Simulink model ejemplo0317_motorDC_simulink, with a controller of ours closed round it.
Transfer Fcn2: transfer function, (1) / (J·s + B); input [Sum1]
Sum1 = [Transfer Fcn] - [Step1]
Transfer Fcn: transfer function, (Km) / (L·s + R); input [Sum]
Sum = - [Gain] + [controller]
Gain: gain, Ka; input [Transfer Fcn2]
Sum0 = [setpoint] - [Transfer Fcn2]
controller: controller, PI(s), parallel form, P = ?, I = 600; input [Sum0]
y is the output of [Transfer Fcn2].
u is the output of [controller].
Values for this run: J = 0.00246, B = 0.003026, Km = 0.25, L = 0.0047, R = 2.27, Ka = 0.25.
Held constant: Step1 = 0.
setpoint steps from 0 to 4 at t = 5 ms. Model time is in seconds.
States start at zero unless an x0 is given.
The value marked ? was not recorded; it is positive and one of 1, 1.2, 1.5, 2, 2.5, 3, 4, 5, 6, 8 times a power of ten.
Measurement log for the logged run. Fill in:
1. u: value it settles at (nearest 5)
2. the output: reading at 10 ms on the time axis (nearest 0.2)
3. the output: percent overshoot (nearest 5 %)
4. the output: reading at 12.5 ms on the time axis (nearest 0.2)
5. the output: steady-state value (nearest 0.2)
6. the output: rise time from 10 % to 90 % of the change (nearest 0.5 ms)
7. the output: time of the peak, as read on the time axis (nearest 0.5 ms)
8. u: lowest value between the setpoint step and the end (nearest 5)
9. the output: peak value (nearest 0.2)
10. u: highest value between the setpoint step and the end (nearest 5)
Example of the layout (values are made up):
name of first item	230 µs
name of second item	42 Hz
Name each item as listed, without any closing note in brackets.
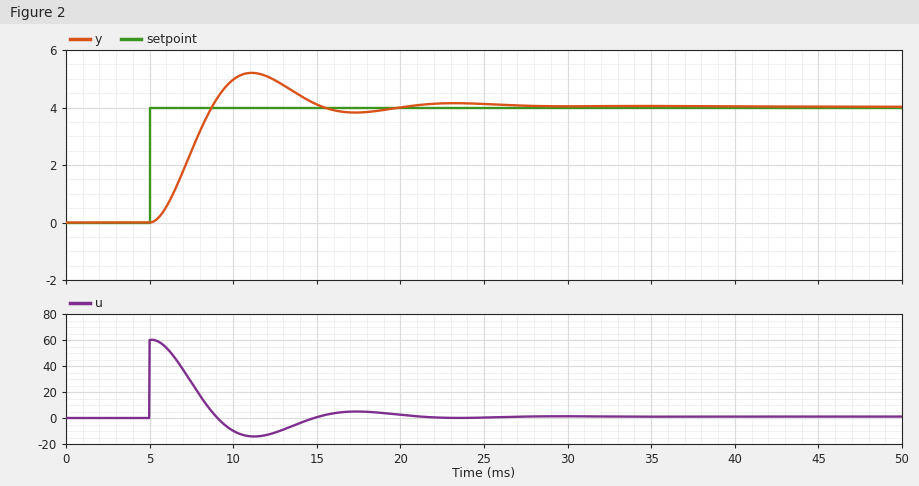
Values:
u: value it settles at	0
the output: reading at 10 ms on the time axis	5.0
the output: percent overshoot	30 %
the output: reading at 12.5 ms on the time axis	5.0
the output: steady-state value	4.0
the output: rise time from 10 % to 90 % of the change	2.5 ms
the output: time of the peak, as read on the time axis	11.0 ms
u: lowest value between the setpoint step and the end	-15
the output: peak value	5.2
u: highest value between the setpoint step and the end	60
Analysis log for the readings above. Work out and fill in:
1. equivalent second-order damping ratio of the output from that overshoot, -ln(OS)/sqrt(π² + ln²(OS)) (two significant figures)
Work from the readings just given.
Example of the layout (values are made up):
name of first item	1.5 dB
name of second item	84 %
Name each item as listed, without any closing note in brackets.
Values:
equivalent second-order damping ratio of the output from that overshoot, -ln(OS)/sqrt(π² + ln²(OS))	0.36
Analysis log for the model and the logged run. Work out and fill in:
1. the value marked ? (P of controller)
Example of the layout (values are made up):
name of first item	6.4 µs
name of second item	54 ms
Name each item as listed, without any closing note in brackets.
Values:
the value marked ?	15
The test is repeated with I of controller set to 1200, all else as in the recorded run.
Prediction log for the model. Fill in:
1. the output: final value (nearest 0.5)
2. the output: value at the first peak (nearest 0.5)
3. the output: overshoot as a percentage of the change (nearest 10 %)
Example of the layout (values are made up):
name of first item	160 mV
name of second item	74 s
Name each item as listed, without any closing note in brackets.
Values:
the output: final value	4.0
the output: value at the first peak	5.5
the output: overshoot as a percentage of the change	40 %
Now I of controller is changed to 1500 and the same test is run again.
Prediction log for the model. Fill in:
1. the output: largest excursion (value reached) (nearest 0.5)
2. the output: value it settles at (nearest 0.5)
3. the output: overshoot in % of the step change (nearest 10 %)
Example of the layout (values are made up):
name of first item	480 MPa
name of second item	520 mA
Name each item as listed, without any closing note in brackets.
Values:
the output: largest excursion (value reached)	5.5
the output: value it settles at	4.0
the output: overshoot in % of the step change	40 %
